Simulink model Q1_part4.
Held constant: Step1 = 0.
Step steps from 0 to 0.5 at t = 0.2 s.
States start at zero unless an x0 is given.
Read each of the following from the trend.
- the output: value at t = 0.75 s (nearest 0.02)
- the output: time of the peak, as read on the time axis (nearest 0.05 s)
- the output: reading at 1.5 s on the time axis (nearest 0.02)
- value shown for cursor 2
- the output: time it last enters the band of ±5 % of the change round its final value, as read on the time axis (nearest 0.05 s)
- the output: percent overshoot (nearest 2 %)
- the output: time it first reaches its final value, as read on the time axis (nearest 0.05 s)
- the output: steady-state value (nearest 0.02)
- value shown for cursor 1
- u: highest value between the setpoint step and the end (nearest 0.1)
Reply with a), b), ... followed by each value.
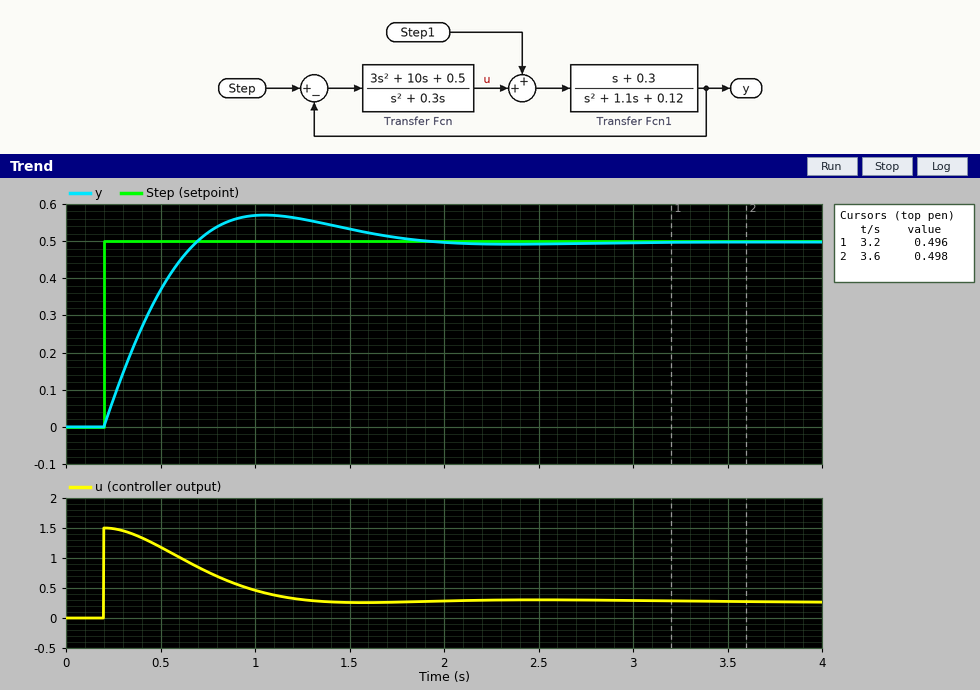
a) 0.52
b) 1.05 s
c) 0.54
d) 0.498
e) 1.60 s
f) 14 %
g) 0.70 s
h) 0.50
i) 0.496
j) 1.5
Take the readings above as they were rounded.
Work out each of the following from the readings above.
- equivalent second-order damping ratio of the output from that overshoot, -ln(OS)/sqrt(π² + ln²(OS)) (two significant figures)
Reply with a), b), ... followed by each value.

a) 0.53
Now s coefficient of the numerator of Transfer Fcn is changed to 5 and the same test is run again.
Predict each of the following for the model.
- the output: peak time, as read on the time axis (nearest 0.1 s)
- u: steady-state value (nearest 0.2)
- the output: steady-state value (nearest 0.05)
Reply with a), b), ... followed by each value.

a) 1.5 s
b) 0.2
c) 0.50
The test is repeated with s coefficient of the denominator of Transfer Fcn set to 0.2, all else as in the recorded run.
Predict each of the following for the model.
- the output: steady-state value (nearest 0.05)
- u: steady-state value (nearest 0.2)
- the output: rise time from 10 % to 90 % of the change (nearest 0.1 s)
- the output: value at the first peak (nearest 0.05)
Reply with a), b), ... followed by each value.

a) 0.50
b) 0.2
c) 0.4 s
d) 0.60
